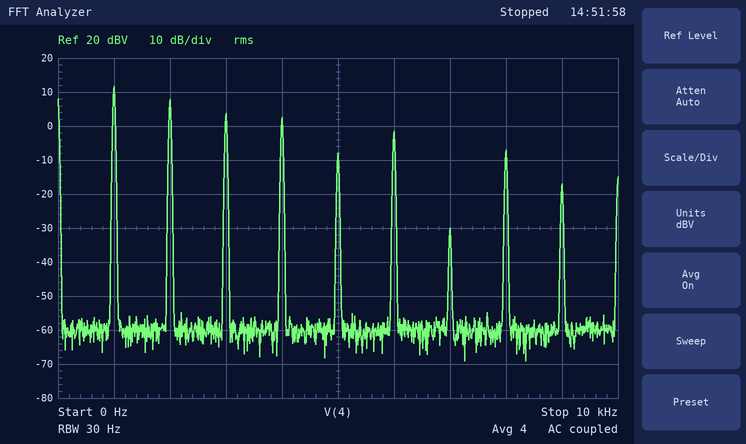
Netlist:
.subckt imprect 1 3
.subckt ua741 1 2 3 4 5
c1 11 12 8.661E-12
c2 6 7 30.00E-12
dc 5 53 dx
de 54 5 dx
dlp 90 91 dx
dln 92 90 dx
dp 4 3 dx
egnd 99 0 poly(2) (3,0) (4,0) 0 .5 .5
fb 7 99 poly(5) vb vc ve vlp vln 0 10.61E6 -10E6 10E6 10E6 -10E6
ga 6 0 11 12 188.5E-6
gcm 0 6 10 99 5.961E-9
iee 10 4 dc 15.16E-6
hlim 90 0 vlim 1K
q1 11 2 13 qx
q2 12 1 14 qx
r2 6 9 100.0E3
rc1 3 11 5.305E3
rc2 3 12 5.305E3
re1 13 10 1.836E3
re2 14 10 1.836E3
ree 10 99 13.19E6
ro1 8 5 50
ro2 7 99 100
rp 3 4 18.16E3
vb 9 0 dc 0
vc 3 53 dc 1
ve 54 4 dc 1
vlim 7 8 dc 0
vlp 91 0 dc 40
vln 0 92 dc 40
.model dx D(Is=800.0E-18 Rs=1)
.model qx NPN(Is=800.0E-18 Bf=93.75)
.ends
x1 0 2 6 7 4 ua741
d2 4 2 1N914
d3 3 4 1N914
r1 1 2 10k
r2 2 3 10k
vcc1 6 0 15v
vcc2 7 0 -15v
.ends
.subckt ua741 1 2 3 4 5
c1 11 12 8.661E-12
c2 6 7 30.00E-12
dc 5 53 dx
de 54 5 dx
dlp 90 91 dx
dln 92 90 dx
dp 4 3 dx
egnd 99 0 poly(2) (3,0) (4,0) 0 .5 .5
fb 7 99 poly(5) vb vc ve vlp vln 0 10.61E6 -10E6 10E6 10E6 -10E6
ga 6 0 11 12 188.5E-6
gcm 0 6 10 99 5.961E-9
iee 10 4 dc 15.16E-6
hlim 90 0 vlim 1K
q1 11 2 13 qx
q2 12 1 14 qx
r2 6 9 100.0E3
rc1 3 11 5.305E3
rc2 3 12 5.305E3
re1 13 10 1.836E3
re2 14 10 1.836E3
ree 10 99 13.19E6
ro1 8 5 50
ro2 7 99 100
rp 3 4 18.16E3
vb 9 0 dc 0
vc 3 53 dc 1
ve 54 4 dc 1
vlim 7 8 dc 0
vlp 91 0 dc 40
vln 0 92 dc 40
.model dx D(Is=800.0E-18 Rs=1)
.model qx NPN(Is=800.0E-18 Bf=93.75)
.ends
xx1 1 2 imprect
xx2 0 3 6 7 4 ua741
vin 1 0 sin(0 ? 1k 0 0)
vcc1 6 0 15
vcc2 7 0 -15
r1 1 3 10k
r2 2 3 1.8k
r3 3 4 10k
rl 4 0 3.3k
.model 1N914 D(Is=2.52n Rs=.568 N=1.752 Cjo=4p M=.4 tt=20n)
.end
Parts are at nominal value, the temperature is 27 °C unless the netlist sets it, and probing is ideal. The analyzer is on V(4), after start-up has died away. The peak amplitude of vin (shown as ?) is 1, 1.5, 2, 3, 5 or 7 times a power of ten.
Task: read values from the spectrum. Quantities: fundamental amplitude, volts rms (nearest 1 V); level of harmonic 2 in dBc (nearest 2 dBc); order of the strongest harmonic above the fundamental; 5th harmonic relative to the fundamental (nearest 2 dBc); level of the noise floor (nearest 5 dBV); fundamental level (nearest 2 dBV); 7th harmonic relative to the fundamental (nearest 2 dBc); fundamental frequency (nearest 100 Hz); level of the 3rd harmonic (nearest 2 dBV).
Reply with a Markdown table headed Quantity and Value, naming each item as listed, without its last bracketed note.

| Quantity | Value |
|---|---|
| fundamental amplitude, volts rms | 4 V |
| level of harmonic 2 in dBc | -4 dBc |
| order of the strongest harmonic above the fundamental | 2 |
| 5th harmonic relative to the fundamental | -20 dBc |
| level of the noise floor | -60 dBV |
| fundamental level | 12 dBV |
| 7th harmonic relative to the fundamental | -42 dBc |
| fundamental frequency | 1.0 kHz |
| level of the 3rd harmonic | 4 dBV |
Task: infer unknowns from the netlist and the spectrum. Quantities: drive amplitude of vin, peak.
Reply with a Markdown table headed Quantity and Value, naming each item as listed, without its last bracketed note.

| Quantity | Value |
|---|---|
| drive amplitude of vin, peak | 7 V |
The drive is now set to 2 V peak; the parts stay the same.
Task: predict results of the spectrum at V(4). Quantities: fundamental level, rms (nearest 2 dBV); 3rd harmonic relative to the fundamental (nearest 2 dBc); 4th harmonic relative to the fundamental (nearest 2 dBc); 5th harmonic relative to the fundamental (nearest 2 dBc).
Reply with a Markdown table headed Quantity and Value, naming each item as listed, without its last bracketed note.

| Quantity | Value |
|---|---|
| fundamental level, rms | 8 dBV |
| 3rd harmonic relative to the fundamental | -58 dBc |
| 4th harmonic relative to the fundamental | -18 dBc |
| 5th harmonic relative to the fundamental | -60 dBc |
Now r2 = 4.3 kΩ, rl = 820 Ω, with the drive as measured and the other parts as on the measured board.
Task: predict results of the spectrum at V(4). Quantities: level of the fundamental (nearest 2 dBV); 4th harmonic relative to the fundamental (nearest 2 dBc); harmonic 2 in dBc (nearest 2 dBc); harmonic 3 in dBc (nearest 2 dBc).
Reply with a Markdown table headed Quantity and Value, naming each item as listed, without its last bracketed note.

| Quantity | Value |
|---|---|
| level of the fundamental | -2 dBV |
| 4th harmonic relative to the fundamental | -4 dBc |
| harmonic 2 in dBc | 10 dBc |
| harmonic 3 in dBc | -54 dBc |
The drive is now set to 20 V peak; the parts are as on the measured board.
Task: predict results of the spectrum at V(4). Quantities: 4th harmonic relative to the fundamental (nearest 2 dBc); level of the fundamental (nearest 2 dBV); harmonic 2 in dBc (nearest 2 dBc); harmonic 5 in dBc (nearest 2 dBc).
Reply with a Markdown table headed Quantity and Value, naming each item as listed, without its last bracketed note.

| Quantity | Value |
|---|---|
| 4th harmonic relative to the fundamental | 8 dBc |
| level of the fundamental | -4 dBV |
| harmonic 2 in dBc | 12 dBc |
| harmonic 5 in dBc | 6 dBc |
